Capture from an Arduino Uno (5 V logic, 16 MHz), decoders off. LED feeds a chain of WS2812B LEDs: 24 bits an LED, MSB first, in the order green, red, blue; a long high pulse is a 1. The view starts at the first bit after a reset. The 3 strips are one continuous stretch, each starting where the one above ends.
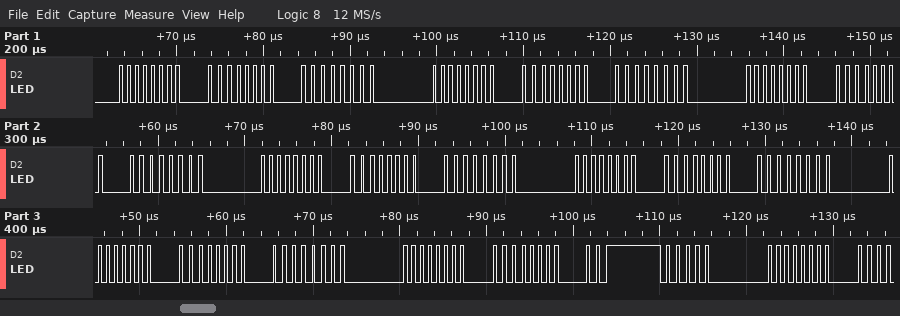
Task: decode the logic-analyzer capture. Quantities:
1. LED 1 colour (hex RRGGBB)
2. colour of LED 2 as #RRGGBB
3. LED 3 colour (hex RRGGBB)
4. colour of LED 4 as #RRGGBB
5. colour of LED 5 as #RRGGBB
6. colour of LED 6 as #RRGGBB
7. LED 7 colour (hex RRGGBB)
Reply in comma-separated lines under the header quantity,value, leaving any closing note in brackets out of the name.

quantity,value
LED 1 colour,#000000
colour of LED 2 as #RRGGBB,#000000
LED 3 colour,#000000
colour of LED 4 as #RRGGBB,#000000
colour of LED 5 as #RRGGBB,#000000
colour of LED 6 as #RRGGBB,#000000
LED 7 colour,#000020
